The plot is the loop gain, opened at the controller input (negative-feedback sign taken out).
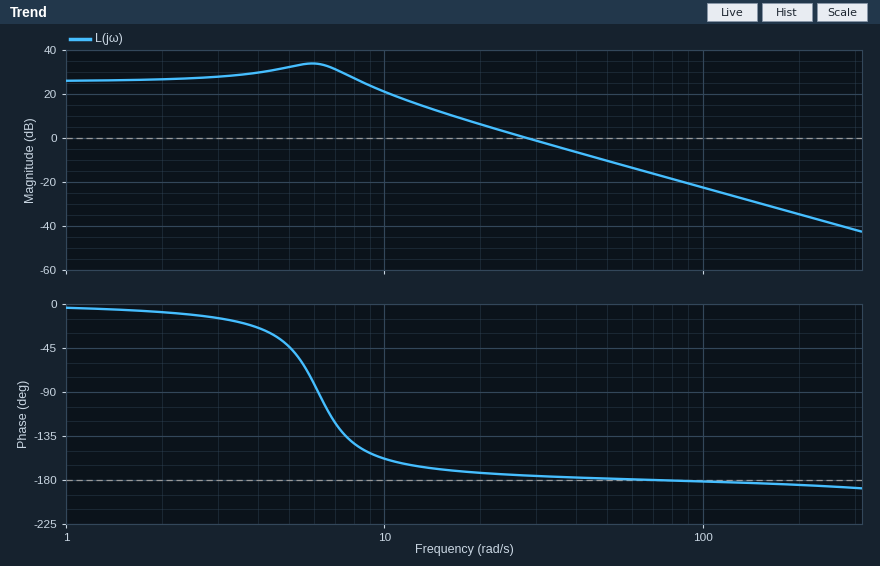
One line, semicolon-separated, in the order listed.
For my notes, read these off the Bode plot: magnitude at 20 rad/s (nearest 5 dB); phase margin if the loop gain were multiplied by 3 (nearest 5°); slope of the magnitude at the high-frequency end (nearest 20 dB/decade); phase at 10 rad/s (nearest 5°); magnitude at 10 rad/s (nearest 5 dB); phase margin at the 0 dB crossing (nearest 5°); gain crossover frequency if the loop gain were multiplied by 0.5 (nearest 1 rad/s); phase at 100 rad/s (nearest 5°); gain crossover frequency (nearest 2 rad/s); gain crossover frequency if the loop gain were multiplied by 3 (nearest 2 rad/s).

5 dB; 0°; -40 dB/decade; -160°; 20 dB; 5°; 20 rad/s; -180°; 28 rad/s; 48 rad/s
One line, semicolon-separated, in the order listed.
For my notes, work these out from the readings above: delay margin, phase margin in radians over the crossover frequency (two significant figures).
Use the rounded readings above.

0.0031 s
